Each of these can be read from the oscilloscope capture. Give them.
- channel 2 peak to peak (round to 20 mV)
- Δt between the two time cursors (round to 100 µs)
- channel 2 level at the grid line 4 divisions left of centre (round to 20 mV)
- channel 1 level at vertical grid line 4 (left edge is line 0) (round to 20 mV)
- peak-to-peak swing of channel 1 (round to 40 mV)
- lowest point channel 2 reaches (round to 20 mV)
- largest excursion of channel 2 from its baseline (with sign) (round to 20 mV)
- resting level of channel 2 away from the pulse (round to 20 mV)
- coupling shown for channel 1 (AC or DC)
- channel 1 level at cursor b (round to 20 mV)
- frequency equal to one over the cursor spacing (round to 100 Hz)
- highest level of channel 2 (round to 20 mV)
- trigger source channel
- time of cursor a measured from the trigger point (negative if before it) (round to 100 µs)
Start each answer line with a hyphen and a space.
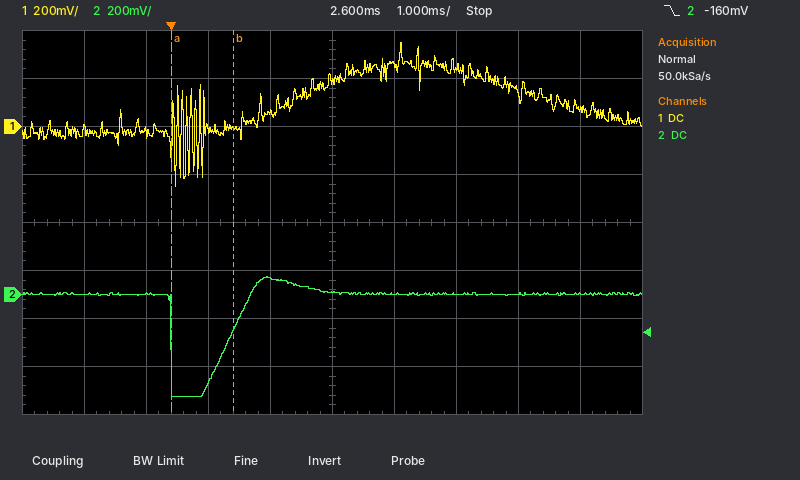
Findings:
- 500 mV
- 1.0 ms
- 0 mV
- 60 mV
- 600 mV
- -420 mV
- -420 mV
- 0 mV
- DC
- 0 mV
- 1.0 kHz
- 80 mV
- channel 2
- 0.0 ms
